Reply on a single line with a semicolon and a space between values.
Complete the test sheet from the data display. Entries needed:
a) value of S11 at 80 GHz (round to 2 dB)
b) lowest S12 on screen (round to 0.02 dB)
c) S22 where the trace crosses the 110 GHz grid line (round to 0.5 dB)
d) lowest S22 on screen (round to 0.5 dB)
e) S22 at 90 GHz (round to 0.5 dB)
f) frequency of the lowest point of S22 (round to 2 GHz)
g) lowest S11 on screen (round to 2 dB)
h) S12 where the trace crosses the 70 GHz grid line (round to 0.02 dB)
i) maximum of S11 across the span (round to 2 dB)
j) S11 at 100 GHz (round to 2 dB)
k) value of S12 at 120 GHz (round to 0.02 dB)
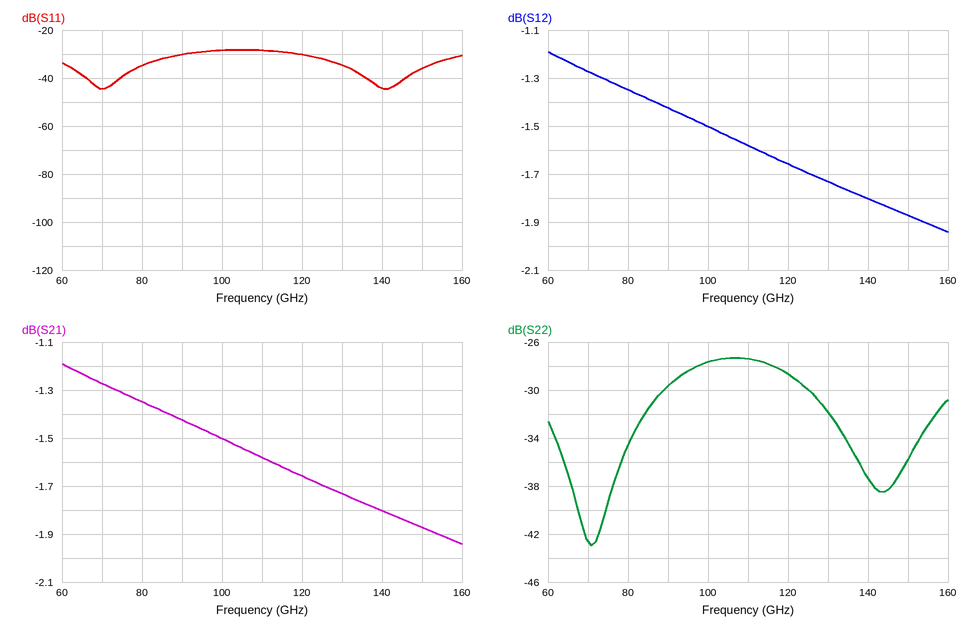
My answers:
-34 dB; -1.94 dB; -27.5 dB; -43.0 dB; -29.5 dB; 70 GHz; -44 dB; -1.28 dB; -28 dB; -28 dB; -1.66 dB
